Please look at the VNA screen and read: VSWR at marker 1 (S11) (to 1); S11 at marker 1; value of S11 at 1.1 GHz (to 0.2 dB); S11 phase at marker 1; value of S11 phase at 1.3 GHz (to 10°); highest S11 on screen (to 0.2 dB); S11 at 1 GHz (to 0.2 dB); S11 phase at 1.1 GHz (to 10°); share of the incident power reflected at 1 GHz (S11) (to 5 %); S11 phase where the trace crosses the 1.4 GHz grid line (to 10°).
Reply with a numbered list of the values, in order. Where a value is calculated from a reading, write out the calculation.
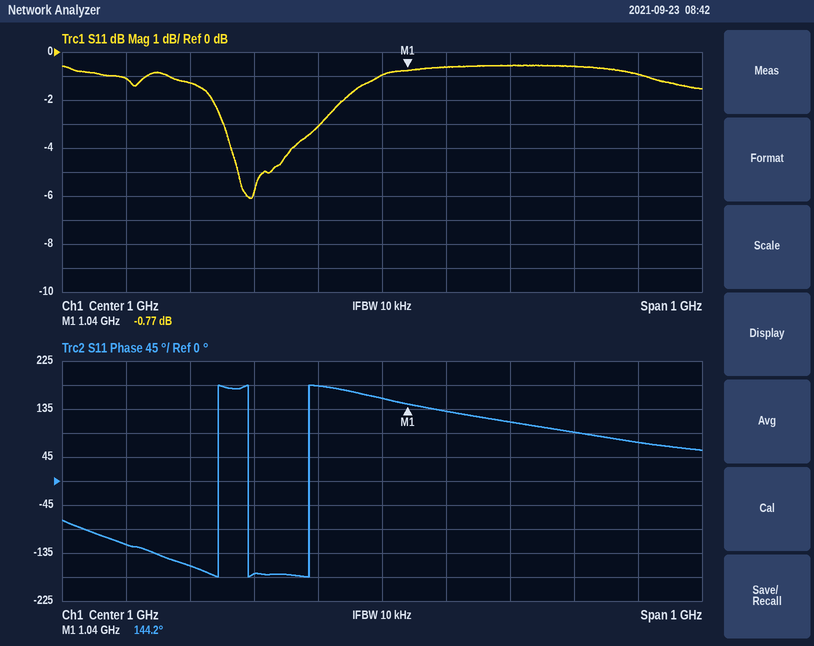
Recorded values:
1. (1 + 0.9152)/(1 − 0.9152) ≈ 23
2. -0.77 dB
3. -0.6 dB
4. 144.2°
5. 90°
6. -0.6 dB
7. -1.0 dB
8. 130°
9. 10^(-1/10) ≈ 79.4 %, so 80 % to the nearest 5 %
10. 70°
